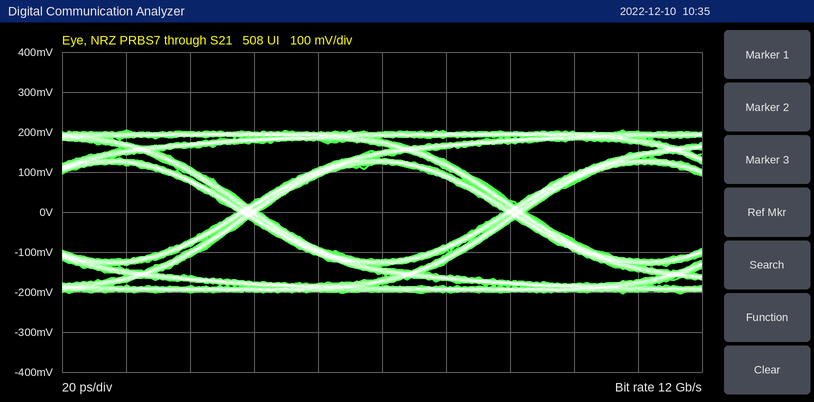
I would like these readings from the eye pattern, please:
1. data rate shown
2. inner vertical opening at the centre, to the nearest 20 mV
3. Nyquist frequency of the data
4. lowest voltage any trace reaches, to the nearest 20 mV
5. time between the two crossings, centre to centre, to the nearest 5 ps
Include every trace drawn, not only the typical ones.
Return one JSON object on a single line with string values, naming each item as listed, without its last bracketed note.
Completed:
{"data rate shown": "12 Gb/s", "inner vertical opening at the centre, to the nearest 20 mV": "240 mV", "Nyquist frequency of the data": "6 GHz", "lowest voltage any trace reaches, to the nearest 20 mV": "-200 mV", "time between the two crossings, centre to centre, to the nearest 5 ps": "85 ps"}
